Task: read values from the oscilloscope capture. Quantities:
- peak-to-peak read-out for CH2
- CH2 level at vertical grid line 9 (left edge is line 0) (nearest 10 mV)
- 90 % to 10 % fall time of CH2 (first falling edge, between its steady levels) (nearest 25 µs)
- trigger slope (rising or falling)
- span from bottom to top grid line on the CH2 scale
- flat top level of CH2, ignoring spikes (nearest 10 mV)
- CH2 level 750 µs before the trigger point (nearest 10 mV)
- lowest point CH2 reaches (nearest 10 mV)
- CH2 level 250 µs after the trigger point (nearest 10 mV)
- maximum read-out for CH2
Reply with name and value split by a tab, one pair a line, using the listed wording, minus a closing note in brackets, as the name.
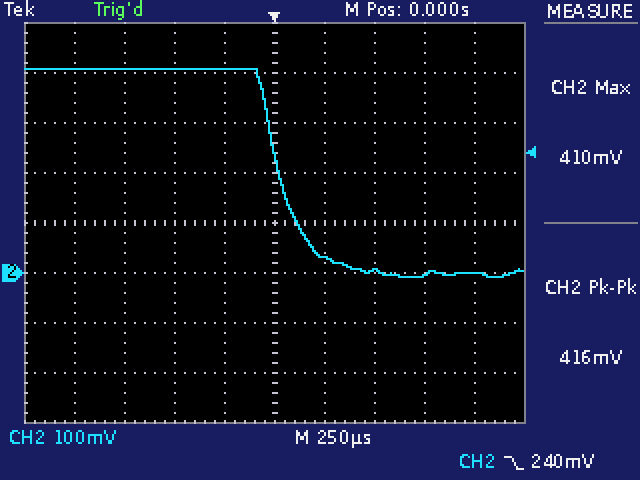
peak-to-peak read-out for CH2	416 mV
CH2 level at vertical grid line 9 (left edge is line 0)	0 mV
90 % to 10 % fall time of CH2 (first falling edge, between its steady levels)	275 µs
trigger slope	falling
span from bottom to top grid line on the CH2 scale	800 mV
flat top level of CH2, ignoring spikes	410 mV
CH2 level 750 µs before the trigger point	410 mV
lowest point CH2 reaches	-10 mV
CH2 level 250 µs after the trigger point	30 mV
maximum read-out for CH2	410 mV
